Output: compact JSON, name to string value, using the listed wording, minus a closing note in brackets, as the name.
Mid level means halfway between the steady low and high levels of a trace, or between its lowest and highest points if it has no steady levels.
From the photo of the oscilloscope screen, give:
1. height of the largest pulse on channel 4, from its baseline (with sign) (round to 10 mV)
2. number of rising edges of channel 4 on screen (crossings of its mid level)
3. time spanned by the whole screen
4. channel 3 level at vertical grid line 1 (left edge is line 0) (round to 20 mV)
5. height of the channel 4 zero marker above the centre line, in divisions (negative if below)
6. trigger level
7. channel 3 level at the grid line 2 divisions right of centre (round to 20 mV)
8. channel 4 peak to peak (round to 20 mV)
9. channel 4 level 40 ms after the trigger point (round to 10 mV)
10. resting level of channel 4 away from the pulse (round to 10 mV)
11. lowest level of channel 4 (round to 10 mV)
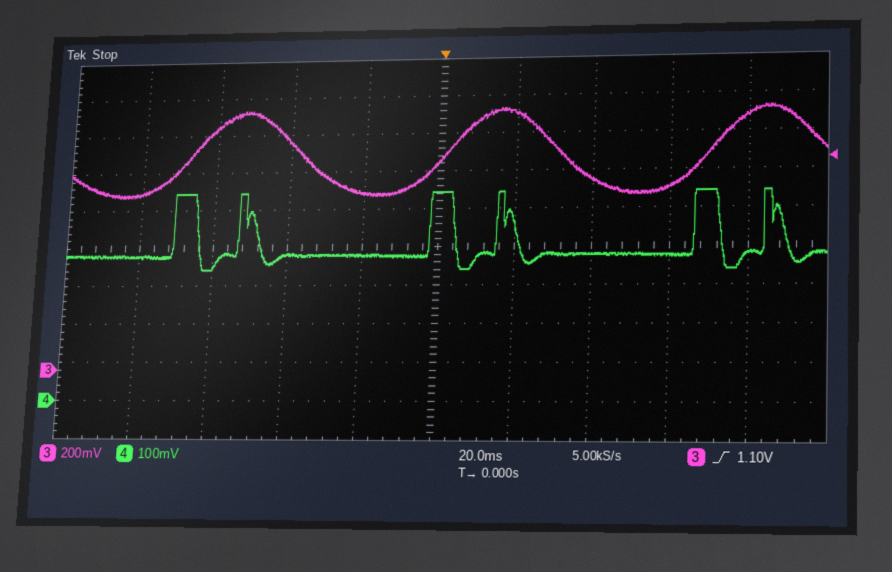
{"height of the largest pulse on channel 4, from its baseline (with sign)": "+170 mV", "number of rising edges of channel 4 on screen": "6", "time spanned by the whole screen": "200 ms", "channel 3 level at vertical grid line 1 (left edge is line 0)": "940 mV", "height of the channel 4 zero marker above the centre line, in divisions": "-4.0 div", "trigger level": "1.10 V", "channel 3 level at the grid line 2 divisions right of centre": "1.00 V", "channel 4 peak to peak": "200 mV", "channel 4 level 40 ms after the trigger point": "380 mV", "resting level of channel 4 away from the pulse": "380 mV", "lowest level of channel 4": "340 mV"}
